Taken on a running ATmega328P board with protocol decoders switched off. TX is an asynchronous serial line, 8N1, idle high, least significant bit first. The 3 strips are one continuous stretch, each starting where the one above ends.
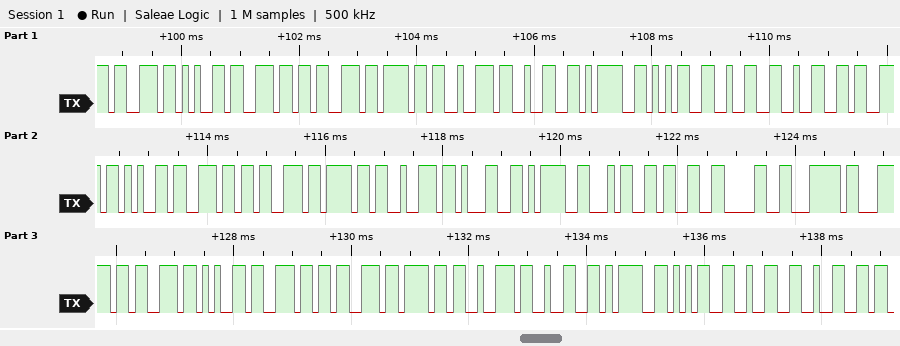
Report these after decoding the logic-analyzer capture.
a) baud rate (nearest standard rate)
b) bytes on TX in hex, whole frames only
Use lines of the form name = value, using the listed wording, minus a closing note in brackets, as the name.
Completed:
baud rate = 9600 baud
bytes on TX in hex, whole frames only = 73 65 6E 73 6F 72 32 3D 35 32 32 73 65 6E 73 6F 72 31 3D 34 33 30 7C 7C 73 65 6E 73 6F 72 32 3D 35 32 32
